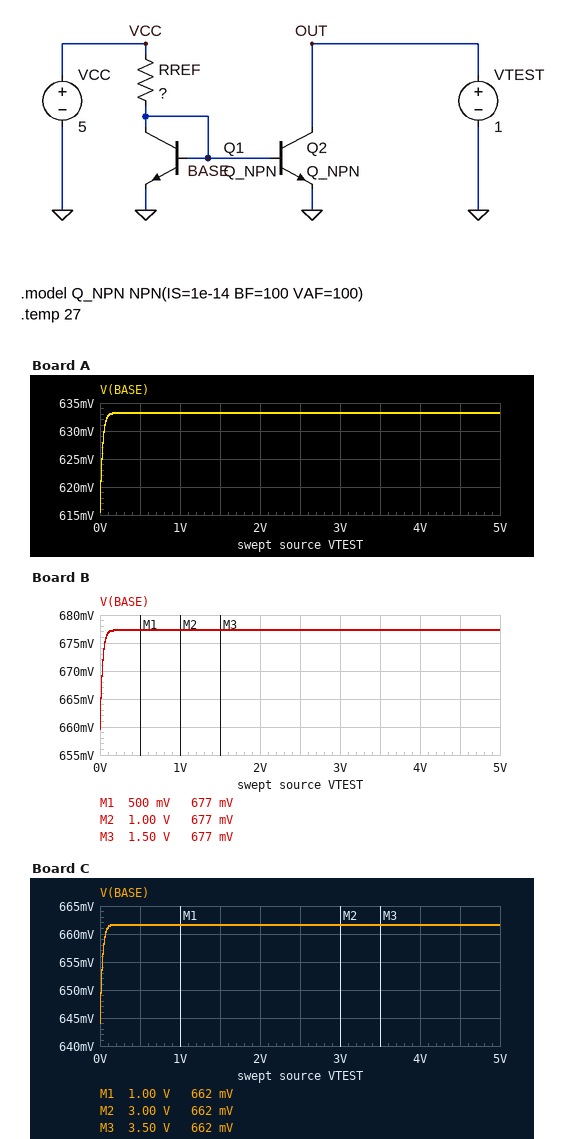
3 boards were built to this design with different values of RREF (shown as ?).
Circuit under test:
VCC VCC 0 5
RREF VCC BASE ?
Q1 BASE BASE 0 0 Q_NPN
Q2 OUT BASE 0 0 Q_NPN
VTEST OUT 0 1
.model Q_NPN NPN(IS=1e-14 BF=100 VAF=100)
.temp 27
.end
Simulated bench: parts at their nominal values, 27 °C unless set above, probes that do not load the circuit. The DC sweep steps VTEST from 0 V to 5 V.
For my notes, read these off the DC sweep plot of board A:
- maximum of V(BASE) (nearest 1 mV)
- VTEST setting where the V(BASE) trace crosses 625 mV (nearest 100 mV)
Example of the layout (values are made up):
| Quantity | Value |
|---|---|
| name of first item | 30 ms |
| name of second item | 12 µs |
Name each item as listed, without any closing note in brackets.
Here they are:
| Quantity | Value |
|---|---|
| maximum of V(BASE) | 633 mV |
| VTEST setting where the V(BASE) trace crosses 625 mV | 0 V |
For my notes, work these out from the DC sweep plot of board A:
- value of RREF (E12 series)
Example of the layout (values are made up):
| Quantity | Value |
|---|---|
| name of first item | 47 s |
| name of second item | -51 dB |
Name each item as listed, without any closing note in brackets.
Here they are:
| Quantity | Value |
|---|---|
| value of RREF | 10 kΩ |
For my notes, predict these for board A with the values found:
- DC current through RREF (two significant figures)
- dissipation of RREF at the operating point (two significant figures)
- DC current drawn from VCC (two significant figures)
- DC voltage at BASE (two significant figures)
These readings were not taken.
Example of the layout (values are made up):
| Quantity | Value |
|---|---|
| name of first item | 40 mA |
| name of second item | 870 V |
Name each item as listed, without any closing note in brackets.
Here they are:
| Quantity | Value |
|---|---|
| DC current through RREF | 440 µA |
| dissipation of RREF at the operating point | 1.9 mW |
| DC current drawn from VCC | 440 µA |
| DC voltage at BASE | 630 mV |
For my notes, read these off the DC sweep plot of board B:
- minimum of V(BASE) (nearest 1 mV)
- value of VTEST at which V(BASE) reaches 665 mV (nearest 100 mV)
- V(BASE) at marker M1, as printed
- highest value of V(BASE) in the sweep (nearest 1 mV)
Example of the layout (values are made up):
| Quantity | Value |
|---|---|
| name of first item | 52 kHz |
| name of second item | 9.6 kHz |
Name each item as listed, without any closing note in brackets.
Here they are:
| Quantity | Value |
|---|---|
| minimum of V(BASE) | 660 mV |
| value of VTEST at which V(BASE) reaches 665 mV | 0 V |
| V(BASE) at marker M1, as printed | 677 mV |
| highest value of V(BASE) in the sweep | 677 mV |
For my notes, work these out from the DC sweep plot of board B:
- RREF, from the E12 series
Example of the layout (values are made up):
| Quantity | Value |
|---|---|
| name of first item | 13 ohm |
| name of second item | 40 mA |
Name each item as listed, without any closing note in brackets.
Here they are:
| Quantity | Value |
|---|---|
| RREF, from the E12 series | 1.8 kΩ |
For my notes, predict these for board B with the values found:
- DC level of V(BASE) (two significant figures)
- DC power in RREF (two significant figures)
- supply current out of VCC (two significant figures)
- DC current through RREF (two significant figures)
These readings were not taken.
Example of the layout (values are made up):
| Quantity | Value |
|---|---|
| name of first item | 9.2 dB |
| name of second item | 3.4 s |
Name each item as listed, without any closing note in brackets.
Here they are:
| Quantity | Value |
|---|---|
| DC level of V(BASE) | 680 mV |
| DC power in RREF | 10 mW |
| supply current out of VCC | 2.4 mA |
| DC current through RREF | 2.4 mA |
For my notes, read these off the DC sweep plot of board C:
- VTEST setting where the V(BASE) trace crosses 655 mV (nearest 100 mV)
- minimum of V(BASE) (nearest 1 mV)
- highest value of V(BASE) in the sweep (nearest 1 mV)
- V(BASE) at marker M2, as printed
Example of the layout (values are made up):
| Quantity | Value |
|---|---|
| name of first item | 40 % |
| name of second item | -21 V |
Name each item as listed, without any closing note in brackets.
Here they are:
| Quantity | Value |
|---|---|
| VTEST setting where the V(BASE) trace crosses 655 mV | 0 V |
| minimum of V(BASE) | 644 mV |
| highest value of V(BASE) in the sweep | 662 mV |
| V(BASE) at marker M2, as printed | 662 mV |
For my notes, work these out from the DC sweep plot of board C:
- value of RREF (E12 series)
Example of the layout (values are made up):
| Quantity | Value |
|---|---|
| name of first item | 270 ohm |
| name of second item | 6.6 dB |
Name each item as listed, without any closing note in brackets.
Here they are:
| Quantity | Value |
|---|---|
| value of RREF | 3.3 kΩ |
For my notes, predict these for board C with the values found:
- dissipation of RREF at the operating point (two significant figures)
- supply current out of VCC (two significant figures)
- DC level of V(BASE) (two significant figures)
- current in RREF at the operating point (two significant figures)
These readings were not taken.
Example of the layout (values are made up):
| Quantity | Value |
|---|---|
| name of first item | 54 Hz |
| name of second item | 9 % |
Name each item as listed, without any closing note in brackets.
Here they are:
| Quantity | Value |
|---|---|
| dissipation of RREF at the operating point | 5.7 mW |
| supply current out of VCC | 1.3 mA |
| DC level of V(BASE) | 660 mV |
| current in RREF at the operating point | 1.3 mA |
